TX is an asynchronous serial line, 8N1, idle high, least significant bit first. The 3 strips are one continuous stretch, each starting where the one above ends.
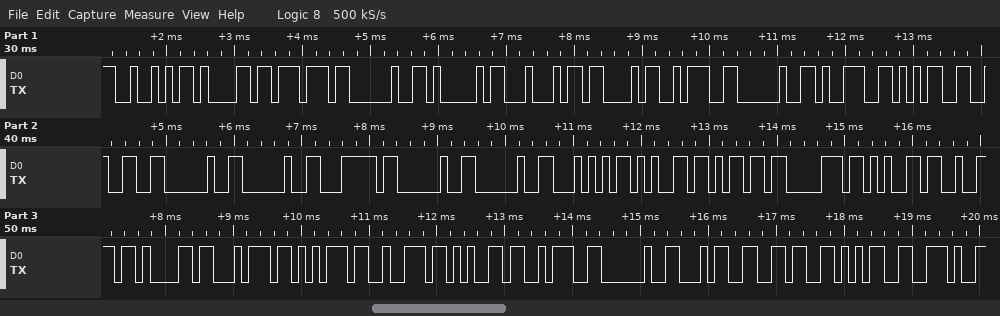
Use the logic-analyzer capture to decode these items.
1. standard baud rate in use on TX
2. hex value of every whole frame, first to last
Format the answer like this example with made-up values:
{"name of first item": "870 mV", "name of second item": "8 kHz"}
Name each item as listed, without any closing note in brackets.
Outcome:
{"standard baud rate in use on TX": "9600 baud", "hex value of every whole frame, first to last": "52 61 77 20 41 44 43 3A 20 39 35 32 20 20 7C 20 20 54 65 6D 70 65 72 61 74 75 72 65 3A 20 34 36 35 2E"}
